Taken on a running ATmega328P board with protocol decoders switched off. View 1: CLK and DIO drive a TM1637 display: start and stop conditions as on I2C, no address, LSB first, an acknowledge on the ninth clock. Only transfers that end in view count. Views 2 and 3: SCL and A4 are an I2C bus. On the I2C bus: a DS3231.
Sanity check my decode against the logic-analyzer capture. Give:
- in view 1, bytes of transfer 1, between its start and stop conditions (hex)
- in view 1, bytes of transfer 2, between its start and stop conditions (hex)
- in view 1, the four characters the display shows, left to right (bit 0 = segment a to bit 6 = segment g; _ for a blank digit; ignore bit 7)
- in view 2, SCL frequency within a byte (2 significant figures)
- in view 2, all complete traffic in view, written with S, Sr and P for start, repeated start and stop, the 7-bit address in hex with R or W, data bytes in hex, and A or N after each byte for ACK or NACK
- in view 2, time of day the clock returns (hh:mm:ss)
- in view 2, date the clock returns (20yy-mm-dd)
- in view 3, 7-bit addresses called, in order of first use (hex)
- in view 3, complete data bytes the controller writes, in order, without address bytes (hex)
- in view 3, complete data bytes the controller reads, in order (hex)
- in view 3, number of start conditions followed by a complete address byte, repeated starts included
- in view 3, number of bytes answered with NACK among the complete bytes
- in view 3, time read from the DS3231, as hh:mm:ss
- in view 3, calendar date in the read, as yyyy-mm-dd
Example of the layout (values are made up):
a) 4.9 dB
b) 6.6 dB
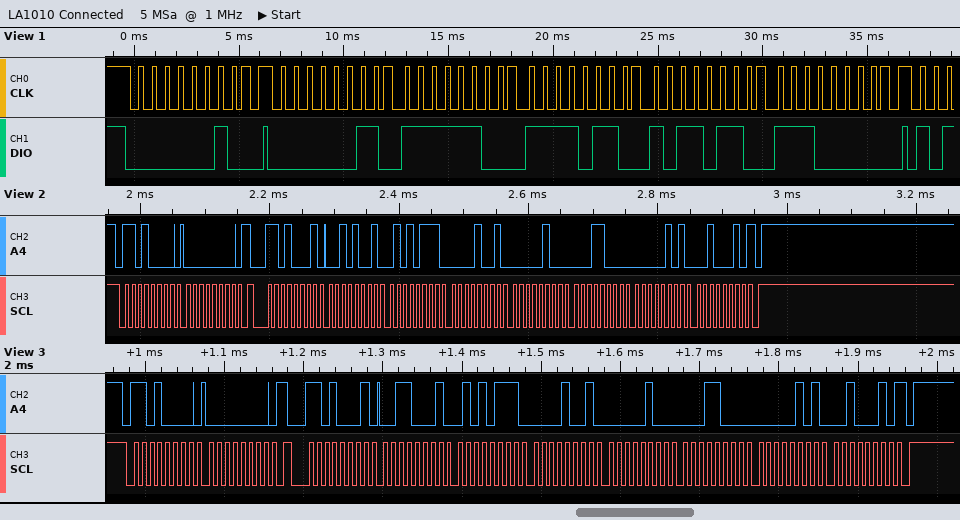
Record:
a) 40
b) C0 3F 6F 6D 07
c) 0957
d) 100 kHz
e) S 68W A 00 A Sr 68R A 29 A 57 A 09 A 04 A 18 A 05 A 22 N P
f) 09:57:29
g) 2022-05-18
h) 0x68
i) 00
j) 31 57 09 04 18 05 22
k) 2
l) 1
m) 09:57:31
n) 2022-05-18
